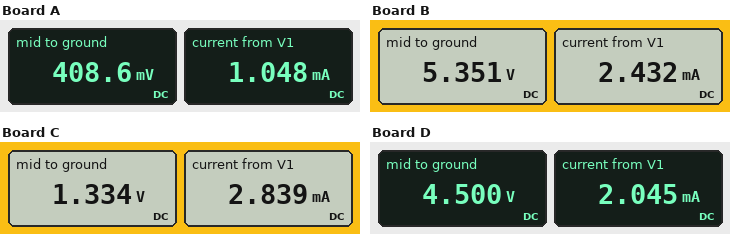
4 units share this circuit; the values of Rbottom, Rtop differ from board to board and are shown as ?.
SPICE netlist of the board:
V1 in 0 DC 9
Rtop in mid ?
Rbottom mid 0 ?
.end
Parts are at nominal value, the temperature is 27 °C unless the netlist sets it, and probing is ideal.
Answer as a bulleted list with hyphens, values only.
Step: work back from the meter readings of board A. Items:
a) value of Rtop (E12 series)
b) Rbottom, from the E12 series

- 8.2 kΩ
- 390 Ω
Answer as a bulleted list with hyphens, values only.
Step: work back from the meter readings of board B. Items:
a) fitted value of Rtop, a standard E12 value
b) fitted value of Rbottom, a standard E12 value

- 1.5 kΩ
- 2.2 kΩ
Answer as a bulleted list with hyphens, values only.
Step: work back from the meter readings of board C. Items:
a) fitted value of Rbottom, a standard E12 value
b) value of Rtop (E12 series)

- 470 Ω
- 2.7 kΩ
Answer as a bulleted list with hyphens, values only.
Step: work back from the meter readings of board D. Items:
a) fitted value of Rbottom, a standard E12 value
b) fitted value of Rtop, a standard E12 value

- 2.2 kΩ
- 2.2 kΩ
